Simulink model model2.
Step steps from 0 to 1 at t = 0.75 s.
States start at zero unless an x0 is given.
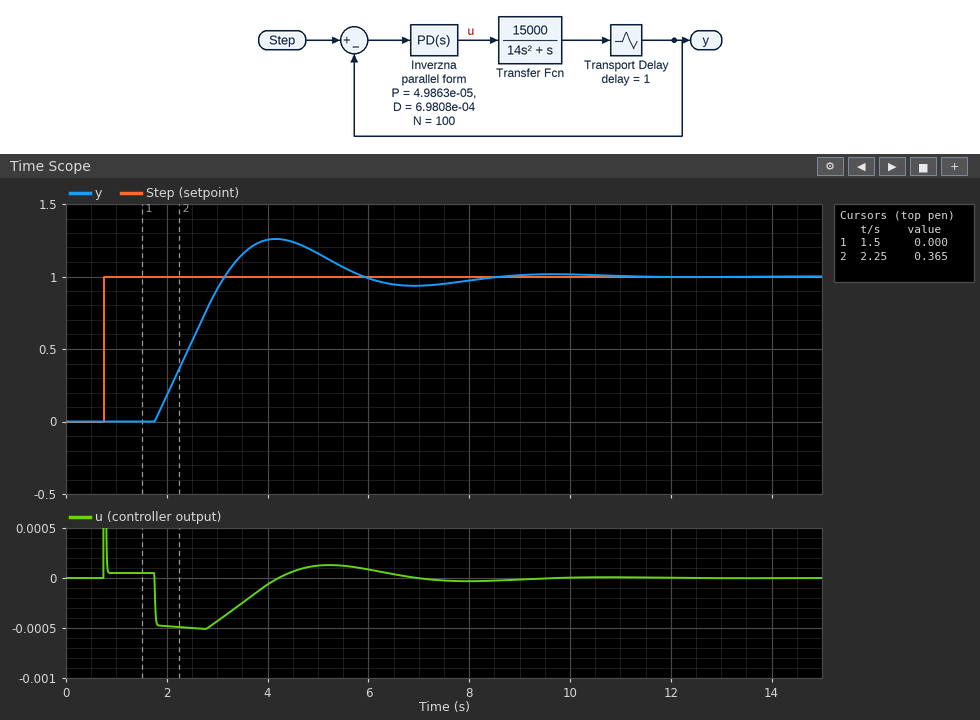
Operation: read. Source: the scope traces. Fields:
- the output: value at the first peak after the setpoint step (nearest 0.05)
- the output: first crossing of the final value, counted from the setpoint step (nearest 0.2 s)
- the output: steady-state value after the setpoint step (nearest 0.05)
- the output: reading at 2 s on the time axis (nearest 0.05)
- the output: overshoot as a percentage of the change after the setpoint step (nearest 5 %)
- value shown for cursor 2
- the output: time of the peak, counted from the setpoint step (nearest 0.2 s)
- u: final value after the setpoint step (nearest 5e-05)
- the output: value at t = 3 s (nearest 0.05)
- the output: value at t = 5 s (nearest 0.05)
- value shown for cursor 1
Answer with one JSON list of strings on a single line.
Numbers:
["1.25", "2.4 s", "1.00", "0.20", "25 %", "0.365", "3.4 s", "0.00000", "0.90", "1.15", "0.000"]
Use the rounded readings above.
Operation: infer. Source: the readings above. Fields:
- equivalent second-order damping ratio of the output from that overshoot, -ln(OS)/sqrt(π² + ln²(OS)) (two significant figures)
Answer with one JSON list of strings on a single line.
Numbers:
["0.40"]
